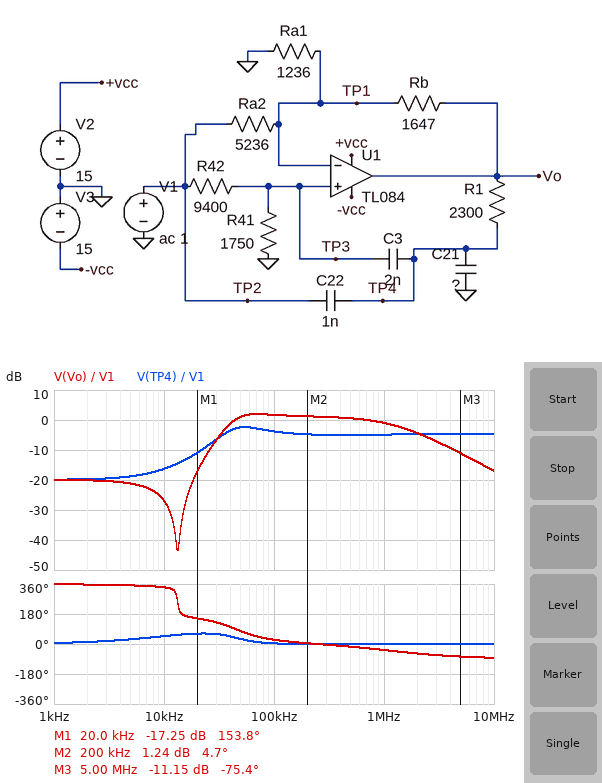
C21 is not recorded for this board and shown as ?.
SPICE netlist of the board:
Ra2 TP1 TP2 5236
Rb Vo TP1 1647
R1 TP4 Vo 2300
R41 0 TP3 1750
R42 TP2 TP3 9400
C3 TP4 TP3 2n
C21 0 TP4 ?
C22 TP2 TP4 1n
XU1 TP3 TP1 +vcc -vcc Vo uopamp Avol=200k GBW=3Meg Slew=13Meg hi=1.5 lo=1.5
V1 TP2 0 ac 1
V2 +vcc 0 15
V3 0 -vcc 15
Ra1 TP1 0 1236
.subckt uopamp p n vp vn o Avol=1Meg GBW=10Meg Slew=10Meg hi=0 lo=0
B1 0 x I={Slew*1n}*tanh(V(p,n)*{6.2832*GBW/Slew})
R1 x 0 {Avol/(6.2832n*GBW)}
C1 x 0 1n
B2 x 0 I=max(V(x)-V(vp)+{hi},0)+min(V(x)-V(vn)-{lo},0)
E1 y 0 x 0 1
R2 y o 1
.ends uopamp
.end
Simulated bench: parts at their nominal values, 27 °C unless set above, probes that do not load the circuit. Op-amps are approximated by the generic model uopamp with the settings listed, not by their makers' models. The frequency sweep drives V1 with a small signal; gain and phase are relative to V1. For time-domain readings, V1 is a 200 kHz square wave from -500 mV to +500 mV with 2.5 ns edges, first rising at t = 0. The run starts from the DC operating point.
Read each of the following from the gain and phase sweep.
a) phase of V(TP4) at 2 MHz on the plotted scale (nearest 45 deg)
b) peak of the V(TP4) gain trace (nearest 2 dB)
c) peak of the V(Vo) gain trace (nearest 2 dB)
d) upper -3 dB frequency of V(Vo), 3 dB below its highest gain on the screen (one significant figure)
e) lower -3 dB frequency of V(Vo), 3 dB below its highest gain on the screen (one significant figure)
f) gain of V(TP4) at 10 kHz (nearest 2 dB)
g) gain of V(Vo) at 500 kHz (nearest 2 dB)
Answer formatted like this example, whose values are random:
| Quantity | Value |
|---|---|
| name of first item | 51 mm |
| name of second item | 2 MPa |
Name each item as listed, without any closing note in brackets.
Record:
| Quantity | Value |
|---|---|
| phase of V(TP4) at 2 MHz on the plotted scale | 0 deg |
| peak of the V(TP4) gain trace | -2 dB |
| peak of the V(Vo) gain trace | 2 dB |
| upper -3 dB frequency of V(Vo), 3 dB below its highest gain on the screen | 1 MHz |
| lower -3 dB frequency of V(Vo), 3 dB below its highest gain on the screen | 40 kHz |
| gain of V(TP4) at 10 kHz | -16 dB |
| gain of V(Vo) at 500 kHz | 0 dB |
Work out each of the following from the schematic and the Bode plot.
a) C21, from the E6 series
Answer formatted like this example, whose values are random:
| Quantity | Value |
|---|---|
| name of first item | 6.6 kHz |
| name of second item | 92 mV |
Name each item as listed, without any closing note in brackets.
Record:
| Quantity | Value |
|---|---|
| C21, from the E6 series | 680 pF |
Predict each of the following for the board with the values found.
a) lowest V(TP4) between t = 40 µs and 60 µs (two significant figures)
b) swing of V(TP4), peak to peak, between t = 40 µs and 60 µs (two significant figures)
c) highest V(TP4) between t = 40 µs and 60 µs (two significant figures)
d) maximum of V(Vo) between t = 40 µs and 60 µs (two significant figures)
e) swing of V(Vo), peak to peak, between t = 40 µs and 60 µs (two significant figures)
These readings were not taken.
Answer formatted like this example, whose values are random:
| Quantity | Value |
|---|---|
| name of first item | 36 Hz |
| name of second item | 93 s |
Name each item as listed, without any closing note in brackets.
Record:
| Quantity | Value |
|---|---|
| lowest V(TP4) between t = 40 µs and 60 µs | -320 mV |
| swing of V(TP4), peak to peak, between t = 40 µs and 60 µs | 640 mV |
| highest V(TP4) between t = 40 µs and 60 µs | 320 mV |
| maximum of V(Vo) between t = 40 µs and 60 µs | 700 mV |
| swing of V(Vo), peak to peak, between t = 40 µs and 60 µs | 1.4 V |
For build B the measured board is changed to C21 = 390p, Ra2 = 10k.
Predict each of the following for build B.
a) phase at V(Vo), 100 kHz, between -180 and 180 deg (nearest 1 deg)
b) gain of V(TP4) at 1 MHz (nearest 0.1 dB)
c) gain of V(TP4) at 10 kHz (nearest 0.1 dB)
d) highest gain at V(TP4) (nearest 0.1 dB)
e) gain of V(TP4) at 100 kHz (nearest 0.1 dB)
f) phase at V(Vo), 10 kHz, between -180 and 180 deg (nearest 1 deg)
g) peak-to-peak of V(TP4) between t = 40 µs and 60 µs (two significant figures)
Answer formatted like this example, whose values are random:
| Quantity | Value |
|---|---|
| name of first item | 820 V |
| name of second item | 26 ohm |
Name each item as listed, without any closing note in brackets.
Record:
| Quantity | Value |
|---|---|
| phase at V(Vo), 100 kHz, between -180 and 180 deg | 22 deg |
| gain of V(TP4) at 1 MHz | -3.3 dB |
| gain of V(TP4) at 10 kHz | -11.7 dB |
| highest gain at V(TP4) | -1.1 dB |
| gain of V(TP4) at 100 kHz | -2.2 dB |
| phase at V(Vo), 10 kHz, between -180 and 180 deg | 13 deg |
| peak-to-peak of V(TP4) between t = 40 µs and 60 µs | 760 mV |
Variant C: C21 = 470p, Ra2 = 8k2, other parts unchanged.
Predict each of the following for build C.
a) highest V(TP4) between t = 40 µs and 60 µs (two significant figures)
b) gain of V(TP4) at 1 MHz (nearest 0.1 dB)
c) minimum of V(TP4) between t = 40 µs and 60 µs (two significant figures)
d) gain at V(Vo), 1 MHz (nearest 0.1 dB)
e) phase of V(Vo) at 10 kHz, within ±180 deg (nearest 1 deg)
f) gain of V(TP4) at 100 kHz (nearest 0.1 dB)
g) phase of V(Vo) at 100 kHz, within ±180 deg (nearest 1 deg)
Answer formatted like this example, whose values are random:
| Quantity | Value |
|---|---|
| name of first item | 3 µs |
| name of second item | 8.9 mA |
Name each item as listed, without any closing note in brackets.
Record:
| Quantity | Value |
|---|---|
| highest V(TP4) between t = 40 µs and 60 µs | 360 mV |
| gain of V(TP4) at 1 MHz | -3.8 dB |
| minimum of V(TP4) between t = 40 µs and 60 µs | -360 mV |
| gain at V(Vo), 1 MHz | 0.8 dB |
| phase of V(Vo) at 10 kHz, within ±180 deg | 11 deg |
| gain of V(TP4) at 100 kHz | -2.7 dB |
| phase of V(Vo) at 100 kHz, within ±180 deg | 23 deg |
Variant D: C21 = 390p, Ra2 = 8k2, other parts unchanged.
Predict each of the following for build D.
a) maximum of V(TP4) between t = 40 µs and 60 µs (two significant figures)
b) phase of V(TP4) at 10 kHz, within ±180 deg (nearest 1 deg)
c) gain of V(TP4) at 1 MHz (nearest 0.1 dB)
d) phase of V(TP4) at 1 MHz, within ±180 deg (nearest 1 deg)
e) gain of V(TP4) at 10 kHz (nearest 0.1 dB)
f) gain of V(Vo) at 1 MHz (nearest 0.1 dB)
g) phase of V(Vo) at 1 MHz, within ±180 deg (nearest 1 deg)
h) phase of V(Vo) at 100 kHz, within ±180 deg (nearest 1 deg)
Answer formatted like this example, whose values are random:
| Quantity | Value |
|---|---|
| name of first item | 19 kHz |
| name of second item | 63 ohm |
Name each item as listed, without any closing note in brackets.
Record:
| Quantity | Value |
|---|---|
| maximum of V(TP4) between t = 40 µs and 60 µs | 380 mV |
| phase of V(TP4) at 10 kHz, within ±180 deg | 30 deg |
| gain of V(TP4) at 1 MHz | -3.3 dB |
| phase of V(TP4) at 1 MHz, within ±180 deg | 2 deg |
| gain of V(TP4) at 10 kHz | -12.7 dB |
| gain of V(Vo) at 1 MHz | 1.3 dB |
| phase of V(Vo) at 1 MHz, within ±180 deg | -35 deg |
| phase of V(Vo) at 100 kHz, within ±180 deg | 23 deg |
